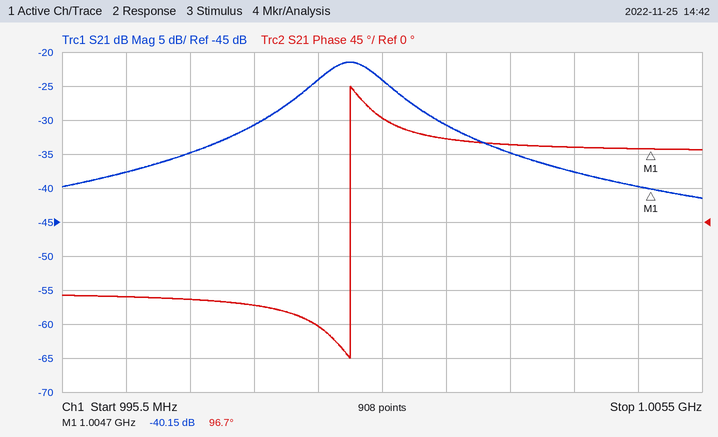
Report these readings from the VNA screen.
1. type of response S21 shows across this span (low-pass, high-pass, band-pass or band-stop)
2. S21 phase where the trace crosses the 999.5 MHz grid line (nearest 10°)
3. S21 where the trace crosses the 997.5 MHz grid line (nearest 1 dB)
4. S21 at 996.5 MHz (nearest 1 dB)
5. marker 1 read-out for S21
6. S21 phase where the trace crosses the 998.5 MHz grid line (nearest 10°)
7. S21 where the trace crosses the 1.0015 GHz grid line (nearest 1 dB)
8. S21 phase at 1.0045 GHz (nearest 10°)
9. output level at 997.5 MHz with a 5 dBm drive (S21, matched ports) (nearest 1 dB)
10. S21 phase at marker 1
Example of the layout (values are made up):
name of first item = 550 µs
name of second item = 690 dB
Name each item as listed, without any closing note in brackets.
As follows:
type of response S21 shows across this span = band-pass
S21 phase where the trace crosses the 999.5 MHz grid line = -140°
S21 where the trace crosses the 997.5 MHz grid line = -35 dB
S21 at 996.5 MHz = -38 dB
marker 1 read-out for S21 = -40.15 dB
S21 phase where the trace crosses the 998.5 MHz grid line = -110°
S21 where the trace crosses the 1.0015 GHz grid line = -31 dB
S21 phase at 1.0045 GHz = 100°
output level at 997.5 MHz with a 5 dBm drive (S21, matched ports) = -30 dBm
S21 phase at marker 1 = 96.7°
